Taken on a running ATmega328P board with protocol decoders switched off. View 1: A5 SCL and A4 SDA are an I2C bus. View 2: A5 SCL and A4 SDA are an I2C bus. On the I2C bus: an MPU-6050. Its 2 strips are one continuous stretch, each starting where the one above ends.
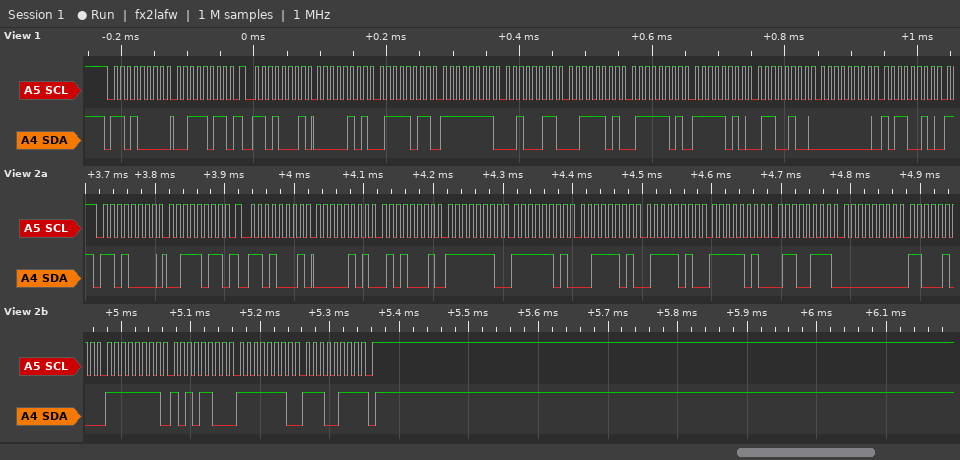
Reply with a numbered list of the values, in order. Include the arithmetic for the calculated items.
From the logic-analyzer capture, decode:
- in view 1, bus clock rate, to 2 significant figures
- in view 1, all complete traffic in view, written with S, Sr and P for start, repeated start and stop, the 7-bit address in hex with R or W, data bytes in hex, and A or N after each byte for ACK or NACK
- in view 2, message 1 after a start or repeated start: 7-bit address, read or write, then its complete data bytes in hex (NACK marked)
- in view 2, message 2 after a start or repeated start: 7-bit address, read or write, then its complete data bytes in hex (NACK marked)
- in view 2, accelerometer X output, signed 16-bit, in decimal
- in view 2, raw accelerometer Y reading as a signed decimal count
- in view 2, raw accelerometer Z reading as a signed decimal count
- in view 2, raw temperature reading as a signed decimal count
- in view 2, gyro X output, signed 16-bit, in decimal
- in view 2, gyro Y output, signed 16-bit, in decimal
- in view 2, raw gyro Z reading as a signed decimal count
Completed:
1. 100 kHz
2. S 68W A 3B A Sr 68R A 05 A 7B A FF A 23 A 3D A 7D A FA A 64 A 00 A B2 A
3. 0x68 write: 3B
4. 0x68 read: 05 51 FE FD 3D 7A FA 67 00 C4 FF AC FE E7 NACK
5. 0x0551 = 1361
6. 0xFEFD = -259
7. 0x3D7A = 15738
8. 0xFA67 = -1433
9. 0x00C4 = 196
10. 0xFFAC = -84
11. 0xFEE7 = -281
